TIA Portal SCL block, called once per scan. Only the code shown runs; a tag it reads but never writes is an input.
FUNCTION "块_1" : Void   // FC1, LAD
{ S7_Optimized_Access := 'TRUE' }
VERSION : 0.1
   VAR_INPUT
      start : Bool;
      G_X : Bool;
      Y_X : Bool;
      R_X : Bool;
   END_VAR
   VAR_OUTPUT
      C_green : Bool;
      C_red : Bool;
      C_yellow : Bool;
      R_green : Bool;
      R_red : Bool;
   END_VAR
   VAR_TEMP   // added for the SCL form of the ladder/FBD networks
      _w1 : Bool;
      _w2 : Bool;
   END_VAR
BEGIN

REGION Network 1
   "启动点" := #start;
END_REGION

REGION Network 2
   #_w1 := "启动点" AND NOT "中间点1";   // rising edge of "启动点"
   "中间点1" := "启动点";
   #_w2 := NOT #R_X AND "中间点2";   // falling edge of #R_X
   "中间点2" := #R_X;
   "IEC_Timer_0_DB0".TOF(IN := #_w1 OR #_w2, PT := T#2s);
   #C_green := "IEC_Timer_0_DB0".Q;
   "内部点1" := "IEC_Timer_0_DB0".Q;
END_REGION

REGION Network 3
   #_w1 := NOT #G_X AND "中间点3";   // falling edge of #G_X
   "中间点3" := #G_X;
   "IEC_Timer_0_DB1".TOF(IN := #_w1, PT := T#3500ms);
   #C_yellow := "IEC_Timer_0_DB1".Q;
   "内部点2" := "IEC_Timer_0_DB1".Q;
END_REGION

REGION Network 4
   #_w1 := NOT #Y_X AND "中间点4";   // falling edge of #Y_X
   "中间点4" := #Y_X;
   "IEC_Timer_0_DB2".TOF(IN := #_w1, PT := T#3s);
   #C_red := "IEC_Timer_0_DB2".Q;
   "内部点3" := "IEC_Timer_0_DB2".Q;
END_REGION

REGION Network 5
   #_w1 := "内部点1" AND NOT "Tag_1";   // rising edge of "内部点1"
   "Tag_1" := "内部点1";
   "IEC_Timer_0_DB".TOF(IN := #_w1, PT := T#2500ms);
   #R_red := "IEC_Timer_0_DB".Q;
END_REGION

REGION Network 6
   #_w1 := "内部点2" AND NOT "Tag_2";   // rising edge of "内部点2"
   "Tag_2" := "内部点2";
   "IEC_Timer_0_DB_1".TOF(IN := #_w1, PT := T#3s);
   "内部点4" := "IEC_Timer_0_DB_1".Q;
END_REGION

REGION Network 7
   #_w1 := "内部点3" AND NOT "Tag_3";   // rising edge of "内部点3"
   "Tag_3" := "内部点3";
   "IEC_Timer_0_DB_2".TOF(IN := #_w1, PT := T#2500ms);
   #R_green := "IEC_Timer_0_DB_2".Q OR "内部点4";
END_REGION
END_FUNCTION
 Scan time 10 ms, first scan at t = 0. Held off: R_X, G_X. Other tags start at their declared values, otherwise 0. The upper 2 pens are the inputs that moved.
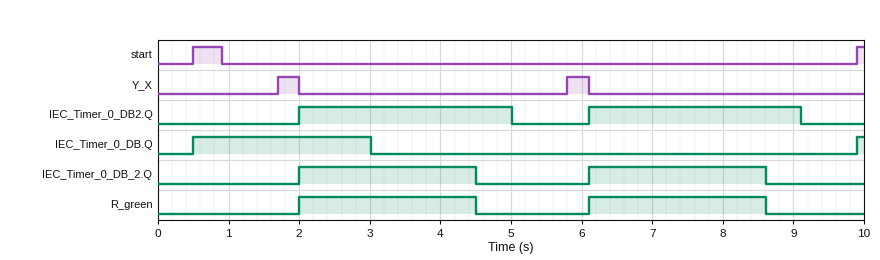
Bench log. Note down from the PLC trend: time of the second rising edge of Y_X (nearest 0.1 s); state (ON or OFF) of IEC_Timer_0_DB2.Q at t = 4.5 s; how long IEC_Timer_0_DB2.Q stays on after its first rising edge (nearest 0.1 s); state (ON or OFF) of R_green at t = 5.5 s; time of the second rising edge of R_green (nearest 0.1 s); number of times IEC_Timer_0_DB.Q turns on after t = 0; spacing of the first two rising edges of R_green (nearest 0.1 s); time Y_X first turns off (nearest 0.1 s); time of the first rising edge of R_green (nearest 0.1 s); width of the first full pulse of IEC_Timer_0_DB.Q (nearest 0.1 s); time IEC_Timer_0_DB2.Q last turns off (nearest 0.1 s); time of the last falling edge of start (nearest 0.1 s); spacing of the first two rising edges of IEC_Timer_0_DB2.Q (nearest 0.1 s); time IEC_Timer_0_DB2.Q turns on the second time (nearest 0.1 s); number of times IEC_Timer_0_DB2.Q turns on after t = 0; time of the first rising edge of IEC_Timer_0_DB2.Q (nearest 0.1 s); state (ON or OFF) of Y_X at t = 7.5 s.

5.8 s
ON
3.0 s
OFF
6.1 s
2
4.1 s
2.0 s
2.0 s
2.5 s
9.1 s
0.9 s
4.1 s
6.1 s
2
2.0 s
OFF
